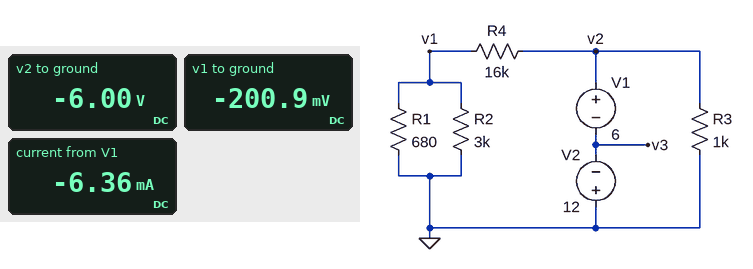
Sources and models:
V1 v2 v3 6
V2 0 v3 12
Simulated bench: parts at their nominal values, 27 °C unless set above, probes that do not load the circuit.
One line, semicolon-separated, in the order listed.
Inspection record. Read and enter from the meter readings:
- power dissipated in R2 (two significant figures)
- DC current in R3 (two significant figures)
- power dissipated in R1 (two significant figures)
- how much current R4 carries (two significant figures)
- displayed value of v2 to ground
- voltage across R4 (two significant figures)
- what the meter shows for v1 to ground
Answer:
13 µW; 6.0 mA; 59 µW; 360 µA; -6.00 V; 5.8 V; -200.9 mV
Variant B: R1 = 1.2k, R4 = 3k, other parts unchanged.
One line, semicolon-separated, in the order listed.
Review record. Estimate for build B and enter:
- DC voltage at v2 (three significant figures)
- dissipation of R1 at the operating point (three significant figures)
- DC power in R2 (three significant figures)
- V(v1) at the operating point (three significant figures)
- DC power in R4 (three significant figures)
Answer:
-6.00 V; 1.48 mW; 593 µW; -1.33 V; 7.26 mW
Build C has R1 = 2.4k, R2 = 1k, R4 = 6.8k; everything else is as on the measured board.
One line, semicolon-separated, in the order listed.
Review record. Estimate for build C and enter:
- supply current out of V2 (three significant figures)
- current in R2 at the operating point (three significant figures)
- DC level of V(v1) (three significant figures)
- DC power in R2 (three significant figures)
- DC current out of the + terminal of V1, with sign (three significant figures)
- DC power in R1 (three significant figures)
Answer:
6.80 mA; 564 µA; -564 mV; 318 µW; -6.80 mA; 133 µW
